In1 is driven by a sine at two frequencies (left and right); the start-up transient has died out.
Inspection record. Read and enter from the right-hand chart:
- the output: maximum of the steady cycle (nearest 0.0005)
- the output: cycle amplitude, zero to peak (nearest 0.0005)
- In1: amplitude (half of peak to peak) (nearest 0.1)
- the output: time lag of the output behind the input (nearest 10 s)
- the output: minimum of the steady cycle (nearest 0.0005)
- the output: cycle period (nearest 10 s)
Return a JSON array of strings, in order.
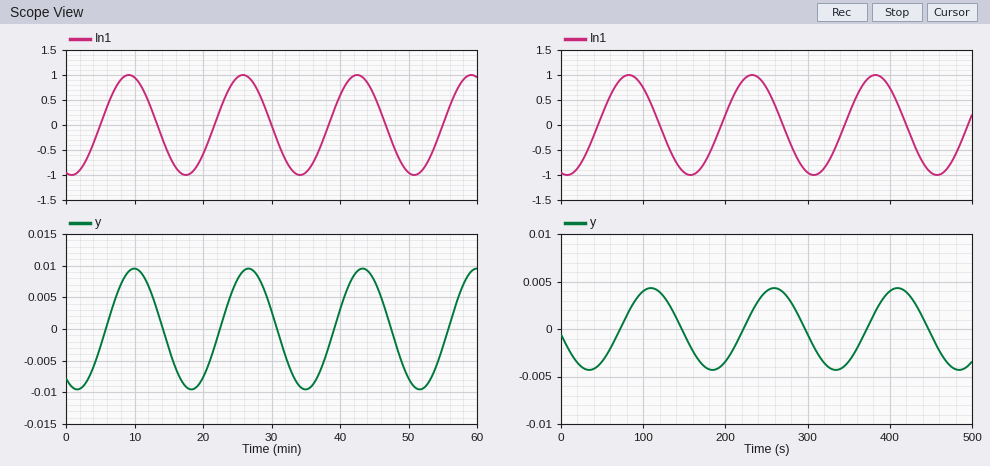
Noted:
["0.0045", "0.0045", "1.0", "30 s", "-0.0045", "150 s"]
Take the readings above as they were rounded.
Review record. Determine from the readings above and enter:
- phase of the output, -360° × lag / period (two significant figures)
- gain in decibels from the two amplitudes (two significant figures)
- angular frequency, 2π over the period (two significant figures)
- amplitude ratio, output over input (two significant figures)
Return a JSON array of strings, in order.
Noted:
["-72°", "-47 dB", "0.042 rad/s", "0.0045"]
